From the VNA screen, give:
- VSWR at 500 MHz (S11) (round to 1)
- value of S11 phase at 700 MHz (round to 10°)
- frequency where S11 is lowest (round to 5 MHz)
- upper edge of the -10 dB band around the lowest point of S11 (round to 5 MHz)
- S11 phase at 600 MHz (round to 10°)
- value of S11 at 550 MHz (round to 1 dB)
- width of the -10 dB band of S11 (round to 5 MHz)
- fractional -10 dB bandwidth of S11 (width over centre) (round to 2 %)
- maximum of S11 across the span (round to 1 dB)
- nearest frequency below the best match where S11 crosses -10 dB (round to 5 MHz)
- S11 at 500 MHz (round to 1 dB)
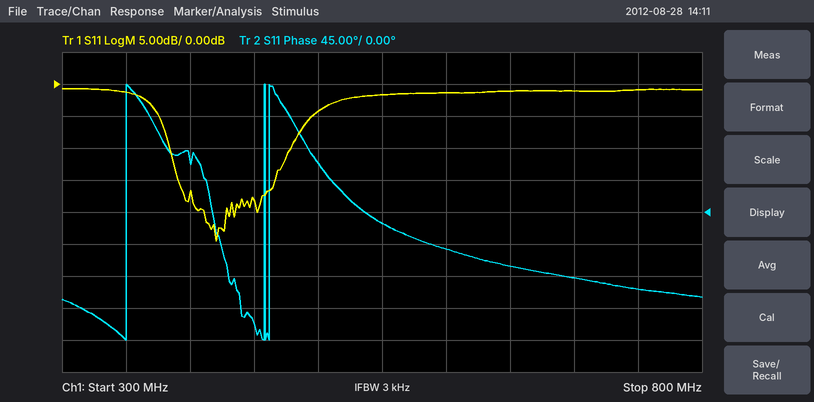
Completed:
4
-90°
420 MHz
480 MHz
-50°
-2 dB
95 MHz
22 %
-1 dB
385 MHz
-4 dB
